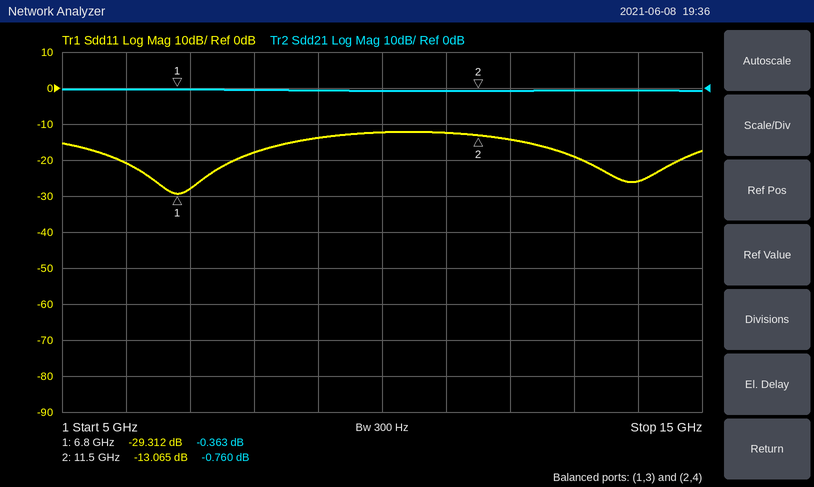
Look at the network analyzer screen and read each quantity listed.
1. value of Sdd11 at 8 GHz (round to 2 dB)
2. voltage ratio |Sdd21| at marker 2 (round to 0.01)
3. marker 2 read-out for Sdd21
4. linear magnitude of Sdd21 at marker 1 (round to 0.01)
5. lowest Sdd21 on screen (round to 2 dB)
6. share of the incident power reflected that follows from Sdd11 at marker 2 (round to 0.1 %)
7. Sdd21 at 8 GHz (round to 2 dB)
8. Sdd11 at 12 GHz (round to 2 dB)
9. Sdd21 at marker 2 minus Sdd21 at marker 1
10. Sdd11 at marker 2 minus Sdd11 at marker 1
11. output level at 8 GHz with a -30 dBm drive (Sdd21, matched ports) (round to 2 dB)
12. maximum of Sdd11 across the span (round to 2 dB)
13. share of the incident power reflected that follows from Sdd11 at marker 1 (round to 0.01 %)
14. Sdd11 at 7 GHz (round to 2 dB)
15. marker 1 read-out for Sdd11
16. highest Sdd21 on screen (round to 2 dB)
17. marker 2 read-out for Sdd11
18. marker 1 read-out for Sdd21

-18 dB
0.92
-0.760 dB
0.96
0 dB
4.9 %
0 dB
-14 dB
-0.397 dB
16.247 dB
-30 dBm
-12 dB
0.12 %
-28 dB
-29.312 dB
0 dB
-13.065 dB
-0.363 dB
